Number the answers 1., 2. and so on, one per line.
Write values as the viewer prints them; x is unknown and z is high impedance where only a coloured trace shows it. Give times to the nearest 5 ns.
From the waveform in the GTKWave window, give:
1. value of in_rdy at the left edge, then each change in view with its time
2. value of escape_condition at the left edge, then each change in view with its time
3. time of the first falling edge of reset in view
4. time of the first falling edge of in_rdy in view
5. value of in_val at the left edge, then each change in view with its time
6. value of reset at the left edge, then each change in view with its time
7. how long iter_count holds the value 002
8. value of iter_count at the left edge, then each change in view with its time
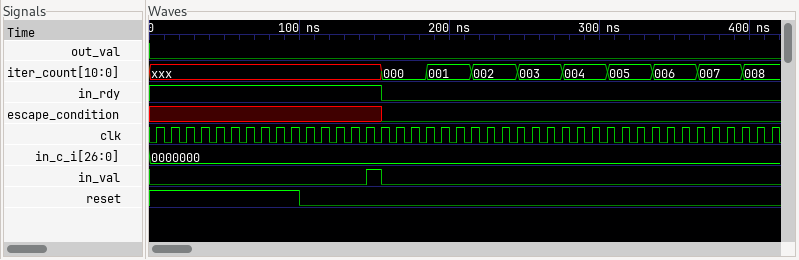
1. 1, 0 at 155 ns
2. x, 0 at 155 ns
3. 100 ns
4. 155 ns
5. 0, 1 at 145 ns, 0 at 155 ns
6. 1, 0 at 100 ns
7. 30 ns
8. xxx, 000 at 155 ns, 001 at 185 ns, 002 at 215 ns, 003 at 245 ns, 004 at 275 ns, 005 at 305 ns, 006 at 335 ns, 007 at 365 ns, 008 at 395 ns
